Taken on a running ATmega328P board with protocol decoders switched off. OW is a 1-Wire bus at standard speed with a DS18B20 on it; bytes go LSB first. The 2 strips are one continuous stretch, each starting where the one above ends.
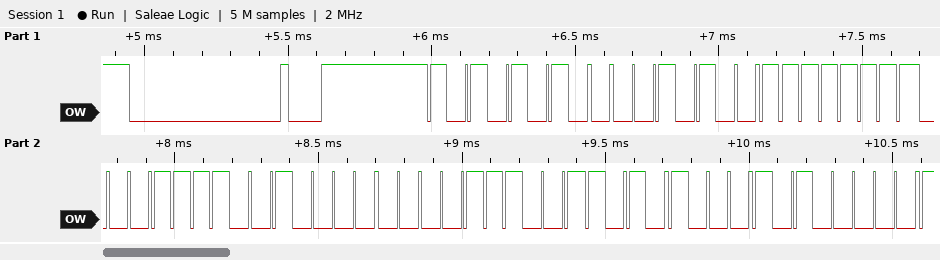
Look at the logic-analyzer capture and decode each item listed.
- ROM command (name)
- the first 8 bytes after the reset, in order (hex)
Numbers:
Match ROM
55 28 FF 78 02 9C 15 05
